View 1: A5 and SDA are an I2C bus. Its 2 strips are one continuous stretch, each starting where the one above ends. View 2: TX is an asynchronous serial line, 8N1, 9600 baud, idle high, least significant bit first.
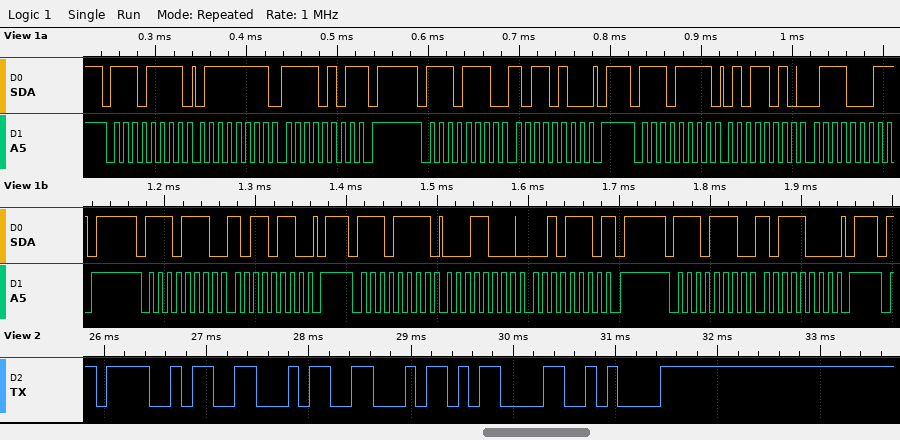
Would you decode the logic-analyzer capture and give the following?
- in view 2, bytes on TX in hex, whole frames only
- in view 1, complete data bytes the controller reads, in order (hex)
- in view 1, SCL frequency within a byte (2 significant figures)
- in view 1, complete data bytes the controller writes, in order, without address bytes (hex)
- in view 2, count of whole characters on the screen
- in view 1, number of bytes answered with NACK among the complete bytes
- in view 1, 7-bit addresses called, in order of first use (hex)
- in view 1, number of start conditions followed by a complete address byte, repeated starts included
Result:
4F 46 46 0D 0A
7F F5 5A 71 18 2E
100 kHz
B4 B6 B8
5
3
0x77
6
